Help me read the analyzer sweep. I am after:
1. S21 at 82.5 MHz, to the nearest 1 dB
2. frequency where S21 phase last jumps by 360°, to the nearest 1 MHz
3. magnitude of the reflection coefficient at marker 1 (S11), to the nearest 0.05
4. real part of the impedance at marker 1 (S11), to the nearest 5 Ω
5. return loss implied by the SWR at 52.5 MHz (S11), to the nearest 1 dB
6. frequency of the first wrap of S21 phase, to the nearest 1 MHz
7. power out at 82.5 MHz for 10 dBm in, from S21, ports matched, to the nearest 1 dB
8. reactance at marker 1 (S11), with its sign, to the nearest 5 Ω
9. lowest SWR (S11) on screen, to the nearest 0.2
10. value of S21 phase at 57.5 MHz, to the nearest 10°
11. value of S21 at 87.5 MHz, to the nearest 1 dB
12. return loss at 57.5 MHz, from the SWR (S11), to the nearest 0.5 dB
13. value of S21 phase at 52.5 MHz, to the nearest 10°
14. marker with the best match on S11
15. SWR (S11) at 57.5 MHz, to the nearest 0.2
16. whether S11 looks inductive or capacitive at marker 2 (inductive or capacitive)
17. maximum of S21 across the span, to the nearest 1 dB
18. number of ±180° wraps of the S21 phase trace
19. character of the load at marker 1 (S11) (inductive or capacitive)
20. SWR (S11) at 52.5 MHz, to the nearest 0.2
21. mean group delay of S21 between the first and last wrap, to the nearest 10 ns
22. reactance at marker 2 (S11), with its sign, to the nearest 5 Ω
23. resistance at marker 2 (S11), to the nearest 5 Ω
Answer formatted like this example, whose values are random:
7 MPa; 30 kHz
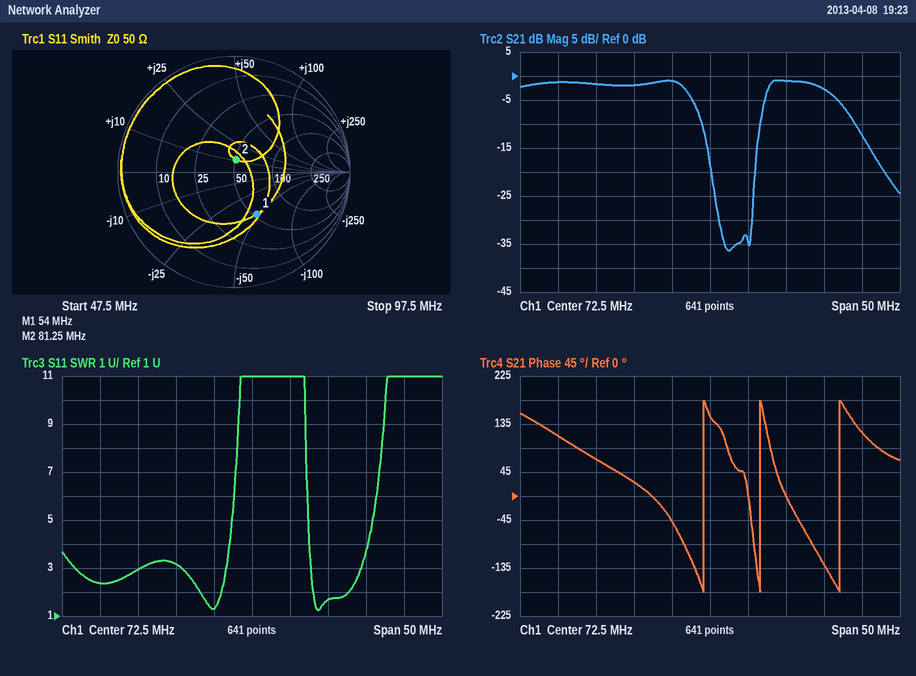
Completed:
-1 dB; 90 MHz; 0.40; 55 Ω; 8 dB; 72 MHz; 9 dBm; -45 Ω; 1.2; 70°; -3 dB; 6.0 dB; 110°; marker 2; 3.0; inductive; -1 dB; 3; capacitive; 2.4; 110 ns; +10 Ω; 50 Ω
